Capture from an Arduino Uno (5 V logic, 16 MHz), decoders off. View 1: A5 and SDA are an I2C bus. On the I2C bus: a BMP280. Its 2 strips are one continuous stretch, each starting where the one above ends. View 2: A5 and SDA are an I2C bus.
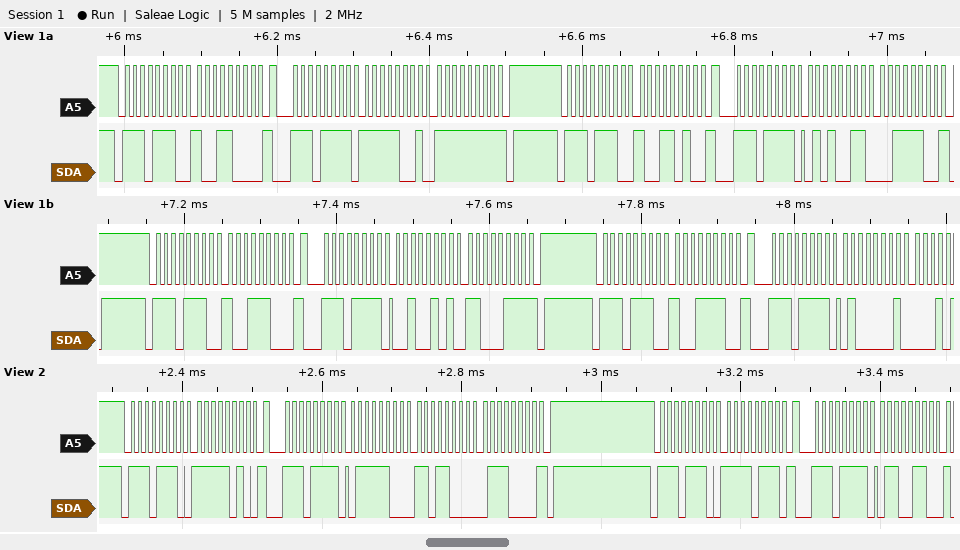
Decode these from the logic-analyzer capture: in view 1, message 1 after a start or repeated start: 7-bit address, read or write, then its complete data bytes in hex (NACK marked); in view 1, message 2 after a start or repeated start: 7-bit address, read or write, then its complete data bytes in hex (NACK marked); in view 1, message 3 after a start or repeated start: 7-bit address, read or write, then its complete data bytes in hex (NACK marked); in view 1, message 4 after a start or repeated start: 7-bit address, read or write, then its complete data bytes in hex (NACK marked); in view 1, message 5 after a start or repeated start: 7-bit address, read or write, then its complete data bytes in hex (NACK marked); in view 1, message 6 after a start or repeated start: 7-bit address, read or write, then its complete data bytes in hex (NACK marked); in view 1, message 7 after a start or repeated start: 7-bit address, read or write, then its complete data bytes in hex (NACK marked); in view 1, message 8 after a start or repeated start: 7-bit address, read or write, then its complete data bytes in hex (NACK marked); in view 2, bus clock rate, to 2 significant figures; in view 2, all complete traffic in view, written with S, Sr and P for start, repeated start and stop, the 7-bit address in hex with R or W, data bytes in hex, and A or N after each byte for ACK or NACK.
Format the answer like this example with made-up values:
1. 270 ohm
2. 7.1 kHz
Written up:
1. 0x77 write: 98
2. 0x77 read: F9 FF NACK
3. 0x77 write: 9A
4. 0x77 read: 53 3C NACK
5. 0x77 write: 9C
6. 0x77 read: 25 C7 NACK
7. 0x77 write: 9E
8. 0x77 read: 41
9. 100 kHz
10. S 77W A FA A Sr 77R A 7C A D8 A 70 N P S 77W A F7 A Sr 77R A 66 A
